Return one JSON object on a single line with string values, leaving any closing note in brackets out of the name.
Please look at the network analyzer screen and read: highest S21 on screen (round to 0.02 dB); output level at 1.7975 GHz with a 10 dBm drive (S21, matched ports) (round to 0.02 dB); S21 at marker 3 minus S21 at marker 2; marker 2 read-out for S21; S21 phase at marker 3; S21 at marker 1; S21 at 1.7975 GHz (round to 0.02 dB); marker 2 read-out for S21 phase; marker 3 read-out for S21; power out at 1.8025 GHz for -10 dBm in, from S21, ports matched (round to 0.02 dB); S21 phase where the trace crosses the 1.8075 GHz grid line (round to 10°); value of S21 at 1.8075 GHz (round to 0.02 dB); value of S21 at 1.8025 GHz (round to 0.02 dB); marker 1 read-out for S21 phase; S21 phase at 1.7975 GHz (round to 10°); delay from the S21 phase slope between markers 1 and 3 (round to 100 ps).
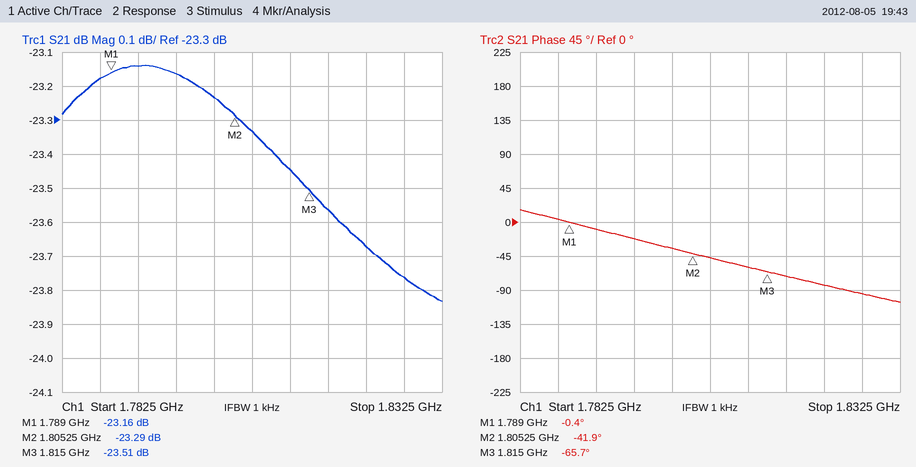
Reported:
{"highest S21 on screen": "-23.14 dB", "output level at 1.7975 GHz with a 10 dBm drive (S21, matched ports)": "-13.16 dBm", "S21 at marker 3 minus S21 at marker 2": "-0.22 dB", "marker 2 read-out for S21": "-23.29 dB", "S21 phase at marker 3": "-65.7°", "S21 at marker 1": "-23.16 dB", "S21 at 1.7975 GHz": "-23.16 dB", "marker 2 read-out for S21 phase": "-41.9°", "marker 3 read-out for S21": "-23.51 dB", "power out at 1.8025 GHz for -10 dBm in, from S21, ports matched": "-33.24 dBm", "S21 phase where the trace crosses the 1.8075 GHz grid line": "-50°", "value of S21 at 1.8075 GHz": "-23.34 dB", "value of S21 at 1.8025 GHz": "-23.24 dB", "marker 1 read-out for S21 phase": "-0.4°", "S21 phase at 1.7975 GHz": "-20°", "delay from the S21 phase slope between markers 1 and 3": "7.0 ns"}
